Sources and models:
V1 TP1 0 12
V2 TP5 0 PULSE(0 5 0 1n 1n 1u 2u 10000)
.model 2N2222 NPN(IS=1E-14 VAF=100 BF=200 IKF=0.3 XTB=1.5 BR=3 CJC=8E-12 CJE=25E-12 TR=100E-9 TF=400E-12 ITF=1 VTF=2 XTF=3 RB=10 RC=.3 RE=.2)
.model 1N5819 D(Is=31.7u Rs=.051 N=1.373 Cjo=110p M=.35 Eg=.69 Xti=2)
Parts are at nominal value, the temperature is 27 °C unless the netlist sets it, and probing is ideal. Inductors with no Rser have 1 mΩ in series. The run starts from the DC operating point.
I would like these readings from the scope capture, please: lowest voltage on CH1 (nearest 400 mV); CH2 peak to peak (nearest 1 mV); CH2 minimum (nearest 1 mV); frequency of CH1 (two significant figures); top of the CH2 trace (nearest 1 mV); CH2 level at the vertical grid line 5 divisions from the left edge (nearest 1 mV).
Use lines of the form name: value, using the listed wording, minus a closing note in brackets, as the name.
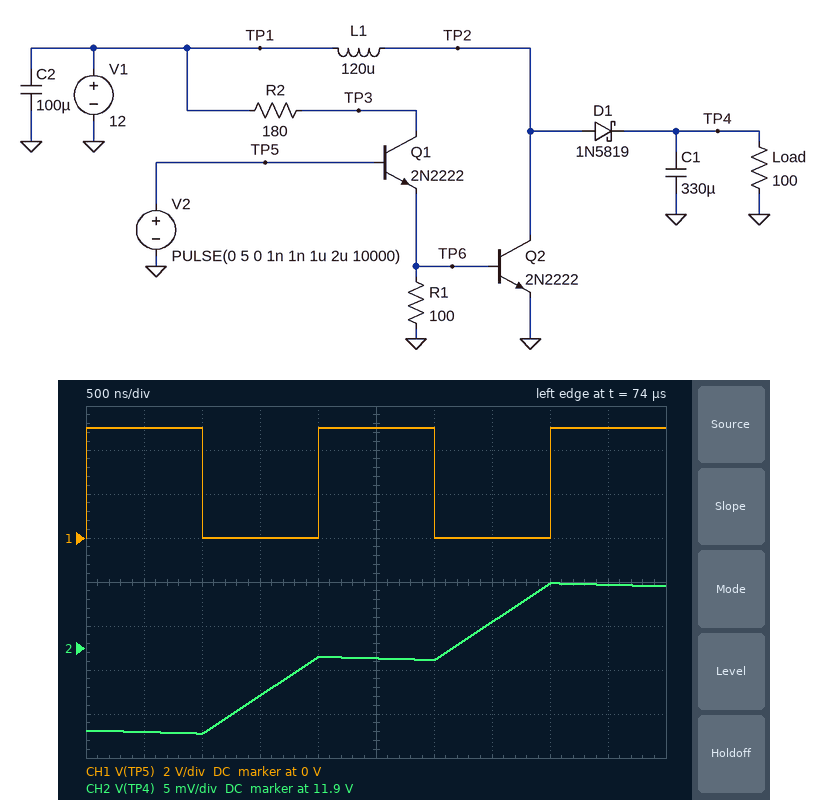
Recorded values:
lowest voltage on CH1: 0 V
CH2 peak to peak: 17 mV
CH2 minimum: 11.895 V
frequency of CH1: 500 kHz
top of the CH2 trace: 11.912 V
CH2 level at the vertical grid line 5 divisions from the left edge: 11.904 V
